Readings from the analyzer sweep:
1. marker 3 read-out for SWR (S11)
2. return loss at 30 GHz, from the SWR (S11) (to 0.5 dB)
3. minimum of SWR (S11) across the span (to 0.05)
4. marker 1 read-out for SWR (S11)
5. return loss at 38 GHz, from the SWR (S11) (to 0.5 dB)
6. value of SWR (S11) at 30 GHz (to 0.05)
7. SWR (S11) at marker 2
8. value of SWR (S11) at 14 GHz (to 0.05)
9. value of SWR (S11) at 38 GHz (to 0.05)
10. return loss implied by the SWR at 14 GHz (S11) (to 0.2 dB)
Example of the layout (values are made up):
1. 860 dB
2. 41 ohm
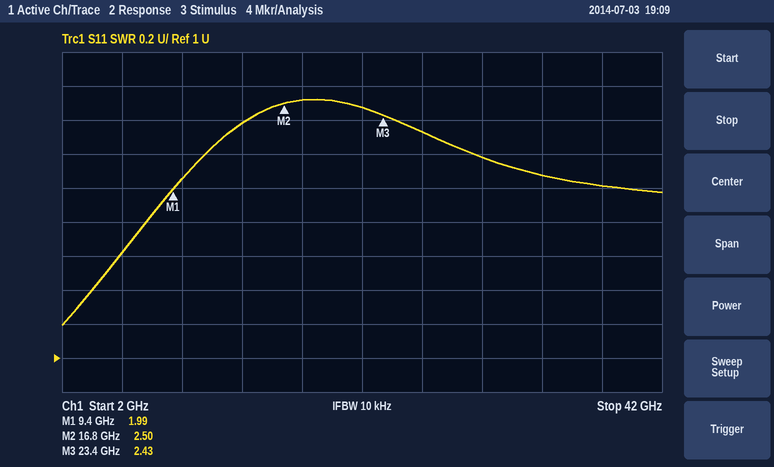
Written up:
1. 2.43
2. 8.5 dB
3. 1.20
4. 1.99
5. 9.5 dB
6. 2.20
7. 2.50
8. 2.40
9. 2.00
10. 7.8 dB
